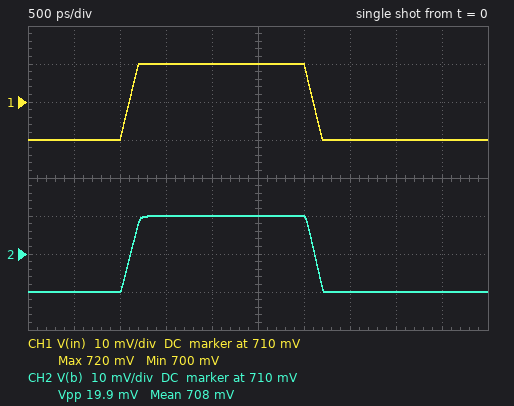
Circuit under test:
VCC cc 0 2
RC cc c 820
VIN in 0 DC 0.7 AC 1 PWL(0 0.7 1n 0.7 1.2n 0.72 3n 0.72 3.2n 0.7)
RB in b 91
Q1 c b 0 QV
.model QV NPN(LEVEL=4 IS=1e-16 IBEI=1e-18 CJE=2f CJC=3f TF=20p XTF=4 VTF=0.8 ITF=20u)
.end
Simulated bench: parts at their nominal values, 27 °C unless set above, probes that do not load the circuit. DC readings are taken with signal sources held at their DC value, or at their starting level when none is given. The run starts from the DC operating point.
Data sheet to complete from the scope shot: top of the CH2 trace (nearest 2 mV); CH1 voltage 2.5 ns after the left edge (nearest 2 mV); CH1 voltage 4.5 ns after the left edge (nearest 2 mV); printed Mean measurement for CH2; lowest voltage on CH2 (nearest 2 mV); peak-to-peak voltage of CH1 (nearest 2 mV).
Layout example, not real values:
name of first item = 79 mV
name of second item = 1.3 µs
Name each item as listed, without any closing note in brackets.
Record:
top of the CH2 trace = 720 mV
CH1 voltage 2.5 ns after the left edge = 720 mV
CH1 voltage 4.5 ns after the left edge = 700 mV
printed Mean measurement for CH2 = 708 mV
lowest voltage on CH2 = 700 mV
peak-to-peak voltage of CH1 = 20 mV
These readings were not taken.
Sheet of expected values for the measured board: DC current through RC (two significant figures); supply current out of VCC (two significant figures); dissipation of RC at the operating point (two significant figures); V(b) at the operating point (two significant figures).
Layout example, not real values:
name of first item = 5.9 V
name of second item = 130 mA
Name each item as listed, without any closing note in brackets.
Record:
DC current through RC = 57 µA
supply current out of VCC = 57 µA
dissipation of RC at the operating point = 2.6 µW
V(b) at the operating point = 700 mV
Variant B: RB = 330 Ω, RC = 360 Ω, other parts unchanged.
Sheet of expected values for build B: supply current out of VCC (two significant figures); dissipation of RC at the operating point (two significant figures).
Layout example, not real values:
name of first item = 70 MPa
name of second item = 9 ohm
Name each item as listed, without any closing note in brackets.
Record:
supply current out of VCC = 56 µA
dissipation of RC at the operating point = 1.1 µW
